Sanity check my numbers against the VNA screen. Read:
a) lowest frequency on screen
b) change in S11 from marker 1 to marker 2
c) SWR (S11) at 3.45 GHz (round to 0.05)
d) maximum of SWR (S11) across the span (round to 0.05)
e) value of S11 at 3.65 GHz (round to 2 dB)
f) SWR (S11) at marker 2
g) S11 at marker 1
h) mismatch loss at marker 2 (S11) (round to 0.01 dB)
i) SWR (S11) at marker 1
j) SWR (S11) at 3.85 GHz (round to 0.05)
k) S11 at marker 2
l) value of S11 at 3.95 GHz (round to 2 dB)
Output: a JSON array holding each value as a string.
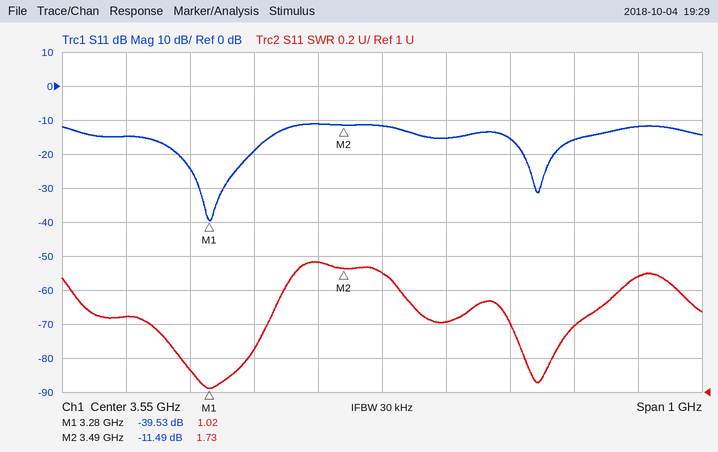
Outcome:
["3.05 GHz", "28.04 dB", "1.75", "1.75", "-16 dB", "1.73", "-39.53 dB", "0.32 dB", "1.02", "1.40", "-11.49 dB", "-12 dB"]
